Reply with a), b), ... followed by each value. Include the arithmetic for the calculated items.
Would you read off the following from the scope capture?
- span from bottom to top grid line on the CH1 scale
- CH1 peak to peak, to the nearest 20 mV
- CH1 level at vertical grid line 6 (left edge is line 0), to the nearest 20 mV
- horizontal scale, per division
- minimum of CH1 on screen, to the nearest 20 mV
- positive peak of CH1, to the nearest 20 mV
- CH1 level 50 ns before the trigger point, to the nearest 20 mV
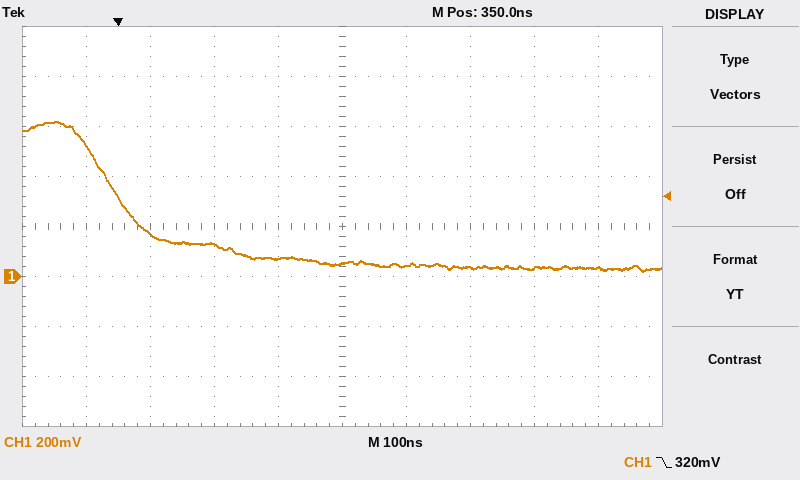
a) 1.6 V
b) 620 mV − (20 mV) = 600 mV
c) 40 mV
d) 100 ns
e) 20 mV
f) 620 mV
g) 520 mV
